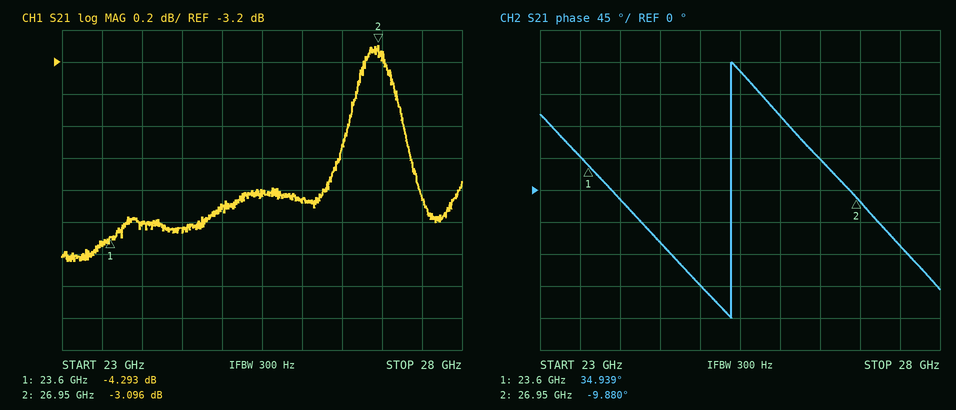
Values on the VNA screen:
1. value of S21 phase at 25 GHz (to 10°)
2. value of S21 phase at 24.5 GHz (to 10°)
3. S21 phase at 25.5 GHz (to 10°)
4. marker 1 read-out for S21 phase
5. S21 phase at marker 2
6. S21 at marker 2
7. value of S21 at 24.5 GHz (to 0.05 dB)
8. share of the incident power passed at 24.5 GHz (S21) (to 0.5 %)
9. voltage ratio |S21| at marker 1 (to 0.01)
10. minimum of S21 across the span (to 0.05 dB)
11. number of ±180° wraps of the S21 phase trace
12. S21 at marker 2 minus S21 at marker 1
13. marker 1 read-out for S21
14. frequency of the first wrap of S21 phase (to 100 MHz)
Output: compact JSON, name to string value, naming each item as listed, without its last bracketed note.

{"value of S21 phase at 25 GHz": "-130°", "value of S21 phase at 24.5 GHz": "-70°", "S21 phase at 25.5 GHz": "170°", "marker 1 read-out for S21 phase": "34.939°", "S21 phase at marker 2": "-9.880°", "S21 at marker 2": "-3.096 dB", "value of S21 at 24.5 GHz": "-4.25 dB", "share of the incident power passed at 24.5 GHz (S21)": "37.5 %", "voltage ratio |S21| at marker 1": "0.61", "minimum of S21 across the span": "-4.45 dB", "number of ±180° wraps of the S21 phase trace": "1", "S21 at marker 2 minus S21 at marker 1": "1.197 dB", "marker 1 read-out for S21": "-4.293 dB", "frequency of the first wrap of S21 phase": "25.4 GHz"}
